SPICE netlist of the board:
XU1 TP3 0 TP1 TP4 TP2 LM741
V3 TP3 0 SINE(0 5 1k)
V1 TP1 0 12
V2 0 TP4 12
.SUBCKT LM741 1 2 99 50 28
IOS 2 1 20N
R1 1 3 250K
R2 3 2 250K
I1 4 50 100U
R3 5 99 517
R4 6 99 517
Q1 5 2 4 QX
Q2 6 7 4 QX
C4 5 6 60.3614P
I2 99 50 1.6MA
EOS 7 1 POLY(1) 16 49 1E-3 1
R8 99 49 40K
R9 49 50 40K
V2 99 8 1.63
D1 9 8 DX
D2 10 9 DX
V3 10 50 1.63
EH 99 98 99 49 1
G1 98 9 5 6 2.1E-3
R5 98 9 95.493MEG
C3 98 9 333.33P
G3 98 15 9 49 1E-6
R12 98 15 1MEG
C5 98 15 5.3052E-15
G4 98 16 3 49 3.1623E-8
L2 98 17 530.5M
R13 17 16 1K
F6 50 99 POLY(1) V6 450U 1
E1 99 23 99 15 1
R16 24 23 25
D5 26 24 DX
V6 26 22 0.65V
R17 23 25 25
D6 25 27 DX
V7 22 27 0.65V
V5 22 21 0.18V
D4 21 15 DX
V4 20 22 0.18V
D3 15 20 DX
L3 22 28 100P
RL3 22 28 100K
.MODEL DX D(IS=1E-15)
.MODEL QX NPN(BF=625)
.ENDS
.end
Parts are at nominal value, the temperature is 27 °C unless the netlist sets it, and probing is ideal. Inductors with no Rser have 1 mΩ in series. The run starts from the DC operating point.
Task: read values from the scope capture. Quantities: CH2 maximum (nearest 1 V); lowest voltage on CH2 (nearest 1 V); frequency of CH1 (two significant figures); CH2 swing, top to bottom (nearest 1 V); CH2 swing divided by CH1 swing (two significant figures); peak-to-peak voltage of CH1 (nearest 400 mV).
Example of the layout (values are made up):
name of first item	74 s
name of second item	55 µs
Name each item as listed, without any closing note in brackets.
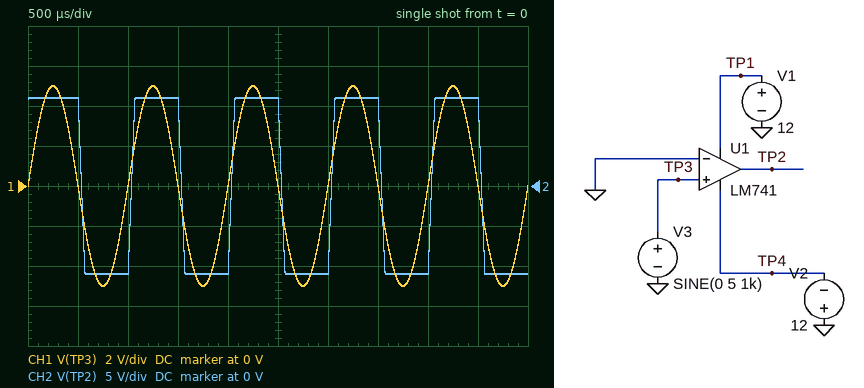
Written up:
CH2 maximum	11 V
lowest voltage on CH2	-11 V
frequency of CH1	1.0 kHz
CH2 swing, top to bottom	22 V
CH2 swing divided by CH1 swing	2.2
peak-to-peak voltage of CH1	10.0 V
